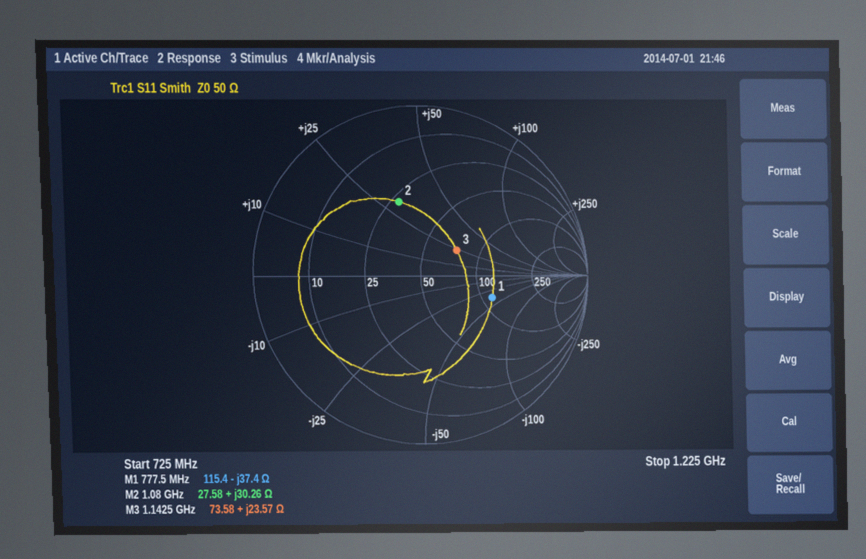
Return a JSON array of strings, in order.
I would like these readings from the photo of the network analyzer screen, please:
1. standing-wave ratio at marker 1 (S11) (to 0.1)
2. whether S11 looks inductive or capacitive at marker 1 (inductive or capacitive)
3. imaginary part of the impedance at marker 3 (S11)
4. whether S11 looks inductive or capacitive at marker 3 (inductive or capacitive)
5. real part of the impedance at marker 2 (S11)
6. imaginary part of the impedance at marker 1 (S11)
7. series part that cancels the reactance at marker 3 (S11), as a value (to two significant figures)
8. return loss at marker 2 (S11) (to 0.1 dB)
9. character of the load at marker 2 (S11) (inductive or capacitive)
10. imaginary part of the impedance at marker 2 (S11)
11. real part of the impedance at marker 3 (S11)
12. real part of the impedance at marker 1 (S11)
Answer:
["2.6", "capacitive", "+23.57 Ω", "inductive", "27.58 Ω", "-37.4 Ω", "5.9 pF", "6.9 dB", "inductive", "+30.26 Ω", "73.58 Ω", "115.4 Ω"]
